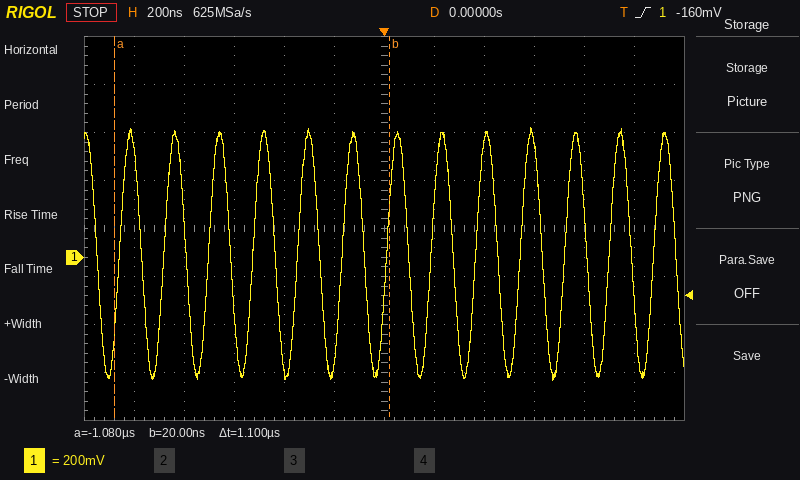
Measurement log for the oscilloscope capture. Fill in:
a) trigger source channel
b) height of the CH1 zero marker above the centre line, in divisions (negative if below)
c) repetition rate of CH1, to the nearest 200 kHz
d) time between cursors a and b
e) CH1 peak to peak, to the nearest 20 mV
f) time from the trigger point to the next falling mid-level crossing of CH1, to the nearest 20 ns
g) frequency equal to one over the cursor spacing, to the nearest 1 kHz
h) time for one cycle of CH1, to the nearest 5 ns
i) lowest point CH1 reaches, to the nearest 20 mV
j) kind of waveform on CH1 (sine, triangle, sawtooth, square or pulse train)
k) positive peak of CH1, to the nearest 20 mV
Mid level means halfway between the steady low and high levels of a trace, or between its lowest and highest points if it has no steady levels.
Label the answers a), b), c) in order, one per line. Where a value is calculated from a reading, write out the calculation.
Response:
a) CH1
b) -0.6 div
c) 1 / 180 ns ≈ 5.6 MHz
d) 1.1 µs
e) 540 mV − (-520 mV) = 1.06 V
f) 100 ns
g) 1 / 1.1 µs ≈ 909 kHz
h) 180 ns
i) -520 mV
j) sine
k) 540 mV
